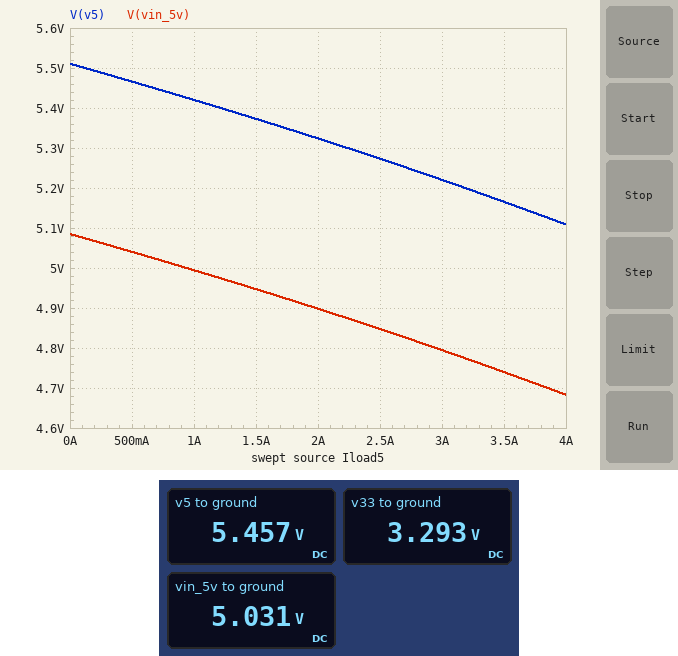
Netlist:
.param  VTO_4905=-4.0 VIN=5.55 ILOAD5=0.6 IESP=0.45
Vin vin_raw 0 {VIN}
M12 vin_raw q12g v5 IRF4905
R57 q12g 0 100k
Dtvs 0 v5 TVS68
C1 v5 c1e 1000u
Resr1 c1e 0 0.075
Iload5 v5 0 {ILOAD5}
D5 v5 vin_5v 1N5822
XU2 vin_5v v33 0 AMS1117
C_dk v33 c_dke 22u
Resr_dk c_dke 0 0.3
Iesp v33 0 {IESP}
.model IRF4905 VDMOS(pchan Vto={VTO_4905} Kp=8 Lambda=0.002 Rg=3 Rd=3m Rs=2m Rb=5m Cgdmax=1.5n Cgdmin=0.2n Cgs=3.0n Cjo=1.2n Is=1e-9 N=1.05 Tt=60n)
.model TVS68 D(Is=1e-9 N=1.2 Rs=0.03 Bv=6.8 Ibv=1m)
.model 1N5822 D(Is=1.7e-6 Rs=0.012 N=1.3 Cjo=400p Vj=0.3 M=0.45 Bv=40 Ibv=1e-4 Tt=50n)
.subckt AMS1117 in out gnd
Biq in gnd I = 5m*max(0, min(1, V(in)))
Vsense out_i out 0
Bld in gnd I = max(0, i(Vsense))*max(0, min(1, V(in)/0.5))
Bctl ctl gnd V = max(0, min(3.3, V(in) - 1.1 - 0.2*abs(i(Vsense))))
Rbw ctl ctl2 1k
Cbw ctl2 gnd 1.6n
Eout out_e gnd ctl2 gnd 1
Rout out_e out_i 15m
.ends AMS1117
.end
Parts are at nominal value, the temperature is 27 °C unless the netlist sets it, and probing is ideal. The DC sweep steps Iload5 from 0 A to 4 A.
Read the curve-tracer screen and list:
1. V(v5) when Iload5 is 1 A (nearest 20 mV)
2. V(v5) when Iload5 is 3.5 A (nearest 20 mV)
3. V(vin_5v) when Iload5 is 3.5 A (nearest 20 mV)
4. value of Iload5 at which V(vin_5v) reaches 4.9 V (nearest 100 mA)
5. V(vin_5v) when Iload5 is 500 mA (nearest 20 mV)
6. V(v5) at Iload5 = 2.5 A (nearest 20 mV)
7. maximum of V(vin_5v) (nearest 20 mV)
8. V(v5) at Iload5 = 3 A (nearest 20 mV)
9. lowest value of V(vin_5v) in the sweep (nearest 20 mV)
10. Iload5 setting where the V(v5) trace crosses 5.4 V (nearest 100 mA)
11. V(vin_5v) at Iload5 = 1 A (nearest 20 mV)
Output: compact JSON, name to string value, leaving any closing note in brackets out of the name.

{"V(v5) when Iload5 is 1 A": "5.42 V", "V(v5) when Iload5 is 3.5 A": "5.16 V", "V(vin_5v) when Iload5 is 3.5 A": "4.74 V", "value of Iload5 at which V(vin_5v) reaches 4.9 V": "2.0 A", "V(vin_5v) when Iload5 is 500 mA": "5.04 V", "V(v5) at Iload5 = 2.5 A": "5.28 V", "maximum of V(vin_5v)": "5.08 V", "V(v5) at Iload5 = 3 A": "5.22 V", "lowest value of V(vin_5v) in the sweep": "4.68 V", "Iload5 setting where the V(v5) trace crosses 5.4 V": "1.2 A", "V(vin_5v) at Iload5 = 1 A": "5.00 V"}
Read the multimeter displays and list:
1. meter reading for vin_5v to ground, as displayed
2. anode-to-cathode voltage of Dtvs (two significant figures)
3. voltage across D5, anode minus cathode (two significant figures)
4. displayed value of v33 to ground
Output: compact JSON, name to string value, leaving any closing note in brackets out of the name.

{"meter reading for vin_5v to ground, as displayed": "5.031 V", "anode-to-cathode voltage of Dtvs": "-5.5 V", "voltage across D5, anode minus cathode": "430 mV", "displayed value of v33 to ground": "3.293 V"}
